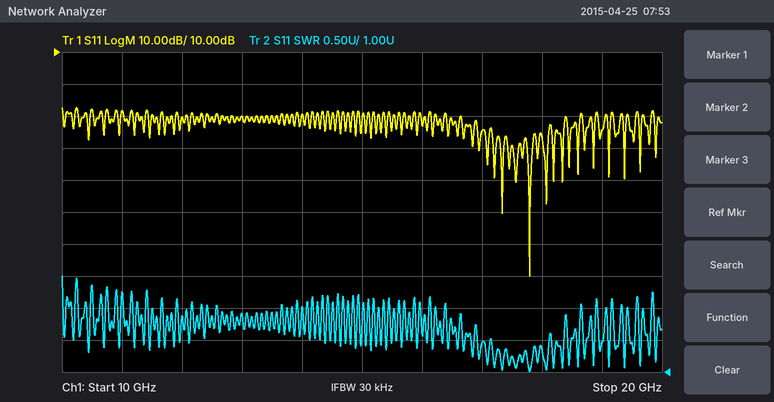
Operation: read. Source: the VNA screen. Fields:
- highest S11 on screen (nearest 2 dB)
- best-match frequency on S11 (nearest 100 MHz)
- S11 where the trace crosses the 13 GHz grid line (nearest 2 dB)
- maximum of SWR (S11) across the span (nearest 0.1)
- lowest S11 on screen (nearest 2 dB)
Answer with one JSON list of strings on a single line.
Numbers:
["-8 dB", "17.8 GHz", "-10 dB", "2.5", "-60 dB"]
